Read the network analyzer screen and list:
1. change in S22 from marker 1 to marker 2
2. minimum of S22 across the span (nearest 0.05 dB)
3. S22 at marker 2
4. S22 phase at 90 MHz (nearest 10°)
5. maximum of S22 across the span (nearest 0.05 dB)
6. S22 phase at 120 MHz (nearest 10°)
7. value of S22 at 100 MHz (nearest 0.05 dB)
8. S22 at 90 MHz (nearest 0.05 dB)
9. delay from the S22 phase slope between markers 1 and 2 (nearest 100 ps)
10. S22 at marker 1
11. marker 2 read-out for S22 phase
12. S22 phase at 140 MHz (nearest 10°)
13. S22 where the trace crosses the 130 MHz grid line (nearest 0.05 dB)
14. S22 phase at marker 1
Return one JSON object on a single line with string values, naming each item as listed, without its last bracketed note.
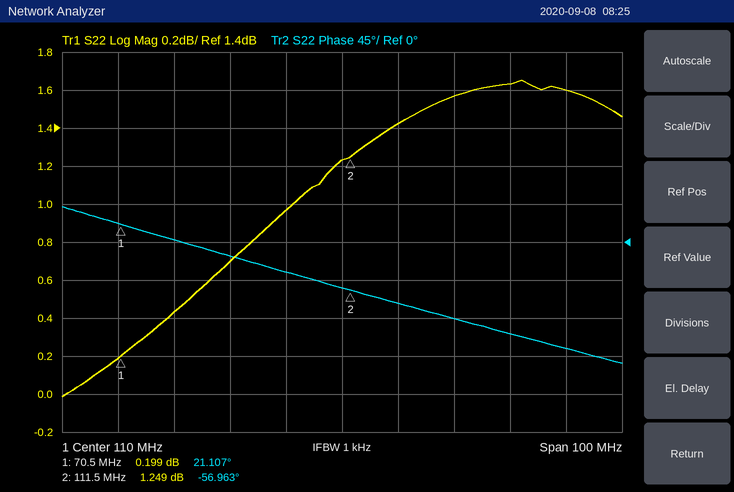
{"change in S22 from marker 1 to marker 2": "1.050 dB", "minimum of S22 across the span": "0.00 dB", "S22 at marker 2": "1.249 dB", "S22 phase at 90 MHz": "-20°", "maximum of S22 across the span": "1.65 dB", "S22 phase at 120 MHz": "-70°", "value of S22 at 100 MHz": "0.95 dB", "S22 at 90 MHz": "0.70 dB", "delay from the S22 phase slope between markers 1 and 2": "5.3 ns", "S22 at marker 1": "0.199 dB", "marker 2 read-out for S22 phase": "-56.963°", "S22 phase at 140 MHz": "-110°", "S22 where the trace crosses the 130 MHz grid line": "1.55 dB", "S22 phase at marker 1": "21.107°"}
